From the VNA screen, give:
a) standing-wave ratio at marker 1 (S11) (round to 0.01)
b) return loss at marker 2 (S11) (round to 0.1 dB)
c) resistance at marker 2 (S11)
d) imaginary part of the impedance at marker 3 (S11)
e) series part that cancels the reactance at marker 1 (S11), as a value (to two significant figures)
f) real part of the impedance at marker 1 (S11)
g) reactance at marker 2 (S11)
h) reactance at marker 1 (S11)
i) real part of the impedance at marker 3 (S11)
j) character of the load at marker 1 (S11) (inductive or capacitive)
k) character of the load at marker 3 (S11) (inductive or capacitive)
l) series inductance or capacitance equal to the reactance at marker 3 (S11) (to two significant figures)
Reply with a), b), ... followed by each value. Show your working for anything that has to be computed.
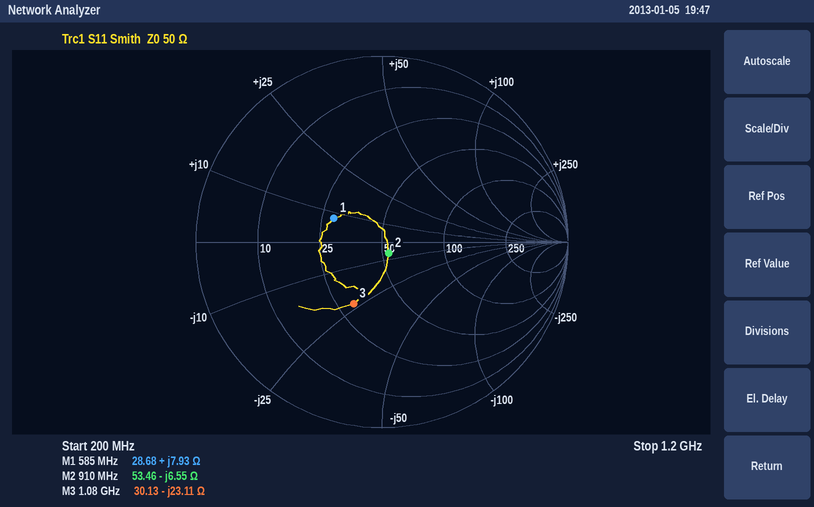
a) 1.81
b) 22.9 dB
c) 53.46 Ω
d) -23.11 Ω
e) C = 1/(2π × 585 MHz × 7.93 Ω) ≈ 34 pF
f) 28.68 Ω
g) -6.55 Ω
h) +7.93 Ω
i) 30.13 Ω
j) inductive
k) capacitive
l) C = 1/(2π × 1.08 GHz × 23.11 Ω) ≈ 6.4 pF
